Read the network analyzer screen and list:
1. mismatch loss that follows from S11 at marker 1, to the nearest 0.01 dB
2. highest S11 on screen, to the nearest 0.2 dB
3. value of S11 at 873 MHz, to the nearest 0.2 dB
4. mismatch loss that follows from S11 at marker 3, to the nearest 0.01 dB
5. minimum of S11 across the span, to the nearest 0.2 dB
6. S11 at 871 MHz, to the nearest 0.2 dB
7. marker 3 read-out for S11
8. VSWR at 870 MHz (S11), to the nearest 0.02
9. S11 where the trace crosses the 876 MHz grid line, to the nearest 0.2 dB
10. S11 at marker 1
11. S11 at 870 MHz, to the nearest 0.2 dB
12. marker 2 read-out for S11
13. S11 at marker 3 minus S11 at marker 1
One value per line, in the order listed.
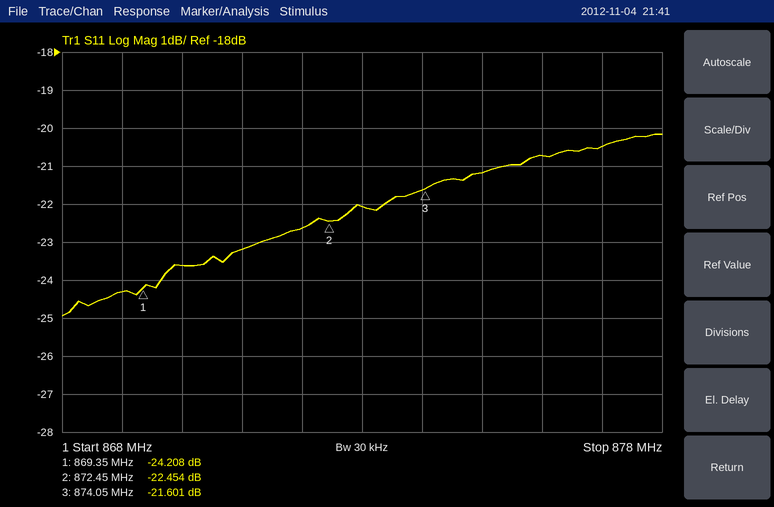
0.02 dB
-20.2 dB
-22.0 dB
0.03 dB
-25.0 dB
-23.2 dB
-21.601 dB
1.14
-20.8 dB
-24.208 dB
-23.6 dB
-22.454 dB
2.607 dB
